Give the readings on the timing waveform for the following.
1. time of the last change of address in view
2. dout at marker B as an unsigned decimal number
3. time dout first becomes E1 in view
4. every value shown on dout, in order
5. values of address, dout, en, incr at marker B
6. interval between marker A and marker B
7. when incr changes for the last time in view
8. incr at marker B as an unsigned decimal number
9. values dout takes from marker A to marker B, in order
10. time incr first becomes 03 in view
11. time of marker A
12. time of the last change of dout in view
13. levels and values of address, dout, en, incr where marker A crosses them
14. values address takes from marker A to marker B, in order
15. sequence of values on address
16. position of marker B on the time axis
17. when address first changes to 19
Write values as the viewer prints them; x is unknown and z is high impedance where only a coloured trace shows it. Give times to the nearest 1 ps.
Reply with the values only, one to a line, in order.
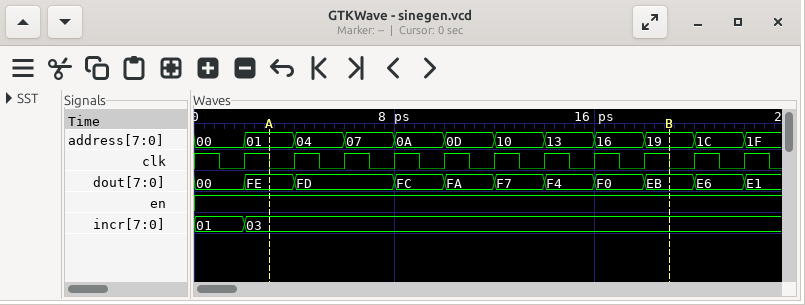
22 ps
235
22 ps
00, FE, FD, FC, FA, F7, F4, F0, EB, E6, E1
address=19, dout=EB, en=1, incr=03
16 ps
2 ps
3
FE, FD, FC, FA, F7, F4, F0, EB
2 ps
3 ps
22 ps
address=01, dout=FE, en=1, incr=03
01, 04, 07, 0A, 0D, 10, 13, 16, 19
00, 01, 04, 07, 0A, 0D, 10, 13, 16, 19, 1C, 1F
19 ps
18 ps
